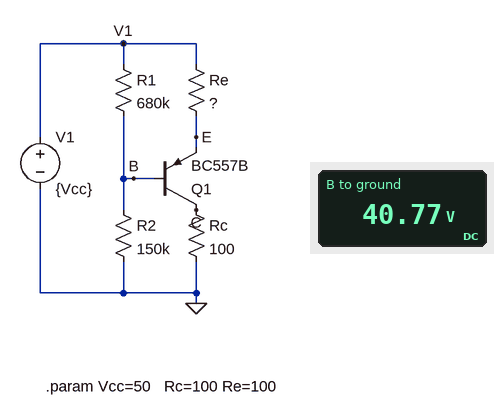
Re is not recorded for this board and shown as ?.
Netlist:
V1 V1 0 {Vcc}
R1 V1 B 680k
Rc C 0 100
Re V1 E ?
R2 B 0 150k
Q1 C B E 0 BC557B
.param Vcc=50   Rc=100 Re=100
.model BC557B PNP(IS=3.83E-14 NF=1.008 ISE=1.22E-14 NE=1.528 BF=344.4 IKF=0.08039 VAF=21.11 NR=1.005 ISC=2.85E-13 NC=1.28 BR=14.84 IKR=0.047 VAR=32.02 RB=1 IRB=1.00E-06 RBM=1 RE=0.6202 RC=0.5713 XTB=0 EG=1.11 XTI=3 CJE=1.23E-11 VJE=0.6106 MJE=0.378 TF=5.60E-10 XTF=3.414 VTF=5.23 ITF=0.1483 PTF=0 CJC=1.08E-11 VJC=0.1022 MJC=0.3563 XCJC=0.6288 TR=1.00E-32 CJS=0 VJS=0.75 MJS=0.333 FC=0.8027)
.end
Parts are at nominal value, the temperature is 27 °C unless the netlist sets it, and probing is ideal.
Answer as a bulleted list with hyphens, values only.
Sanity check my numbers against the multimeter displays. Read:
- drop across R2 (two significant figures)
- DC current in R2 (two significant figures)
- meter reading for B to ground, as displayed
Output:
- 41 V
- 270 µA
- 40.77 V
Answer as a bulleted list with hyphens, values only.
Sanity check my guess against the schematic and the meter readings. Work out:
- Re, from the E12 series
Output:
- 68 Ω
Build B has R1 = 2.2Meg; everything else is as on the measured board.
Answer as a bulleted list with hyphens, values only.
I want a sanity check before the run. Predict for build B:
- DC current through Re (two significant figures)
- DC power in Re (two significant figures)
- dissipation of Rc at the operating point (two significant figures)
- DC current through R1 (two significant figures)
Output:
- 130 mA
- 1.1 W
- 1.6 W
- 4.3 µA
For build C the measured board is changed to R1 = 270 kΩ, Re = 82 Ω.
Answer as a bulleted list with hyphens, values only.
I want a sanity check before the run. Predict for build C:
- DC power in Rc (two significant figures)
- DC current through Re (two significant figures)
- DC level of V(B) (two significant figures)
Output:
- 1.3 W
- 110 mA
- 40 V
